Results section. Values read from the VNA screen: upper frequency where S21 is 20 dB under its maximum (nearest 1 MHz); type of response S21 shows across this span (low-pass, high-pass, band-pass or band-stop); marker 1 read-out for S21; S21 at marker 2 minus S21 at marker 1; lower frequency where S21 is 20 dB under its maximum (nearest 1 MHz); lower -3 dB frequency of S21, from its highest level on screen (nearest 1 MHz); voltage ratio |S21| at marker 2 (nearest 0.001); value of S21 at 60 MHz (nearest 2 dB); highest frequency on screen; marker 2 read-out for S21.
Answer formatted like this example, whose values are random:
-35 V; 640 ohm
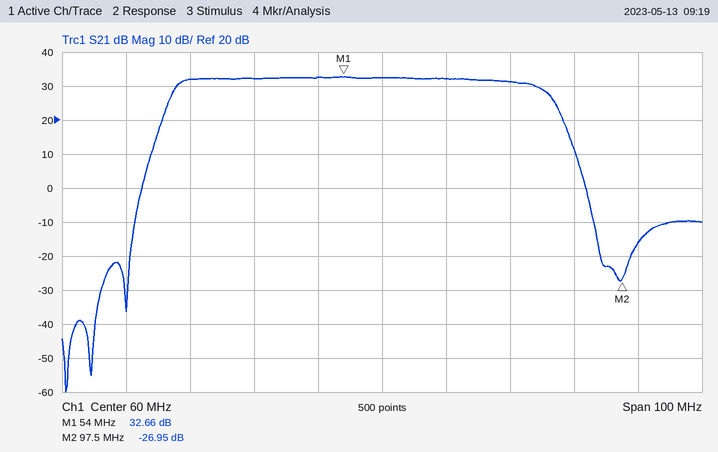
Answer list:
90 MHz; band-pass; 32.66 dB; -59.61 dB; 24 MHz; 28 MHz; 0.045; 32 dB; 110 MHz; -26.95 dB
